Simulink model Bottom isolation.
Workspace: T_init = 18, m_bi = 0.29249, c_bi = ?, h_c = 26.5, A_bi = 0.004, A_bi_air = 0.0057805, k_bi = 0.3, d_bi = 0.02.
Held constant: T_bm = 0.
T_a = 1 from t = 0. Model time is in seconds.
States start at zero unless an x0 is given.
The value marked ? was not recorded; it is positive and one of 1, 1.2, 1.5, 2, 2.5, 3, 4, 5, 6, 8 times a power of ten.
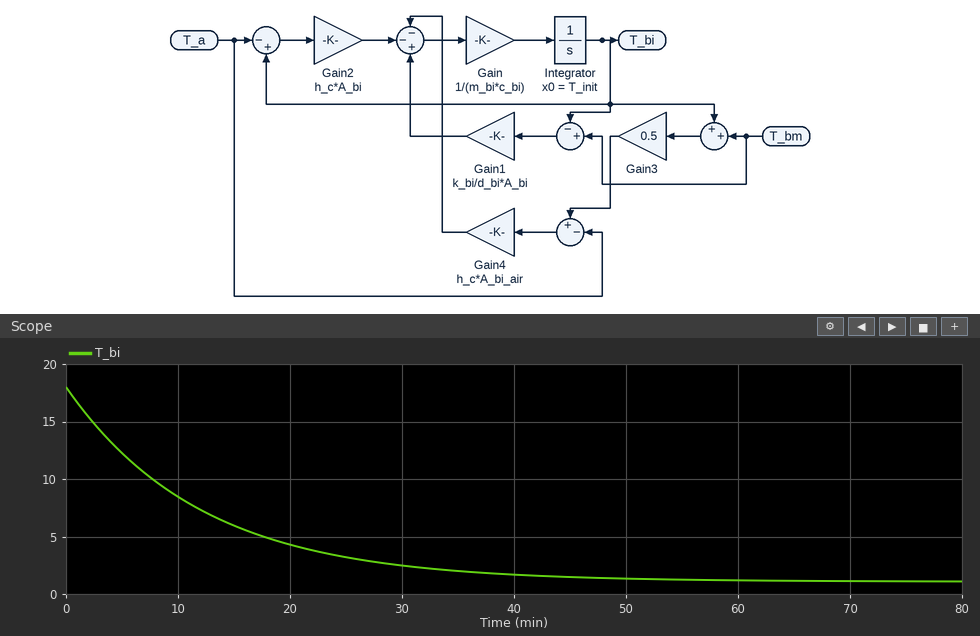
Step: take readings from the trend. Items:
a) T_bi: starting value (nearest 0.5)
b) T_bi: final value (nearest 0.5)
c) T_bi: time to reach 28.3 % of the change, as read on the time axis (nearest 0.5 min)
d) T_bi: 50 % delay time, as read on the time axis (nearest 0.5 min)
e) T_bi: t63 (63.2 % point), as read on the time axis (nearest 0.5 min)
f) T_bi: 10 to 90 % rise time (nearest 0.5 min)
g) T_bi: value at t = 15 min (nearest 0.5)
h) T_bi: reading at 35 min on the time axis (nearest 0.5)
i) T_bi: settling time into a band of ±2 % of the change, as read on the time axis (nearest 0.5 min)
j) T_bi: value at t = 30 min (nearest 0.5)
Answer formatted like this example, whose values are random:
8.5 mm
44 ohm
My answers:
18.0
1.0
4.0 min
8.5 min
12.0 min
26.5 min
6.0
2.0
47.0 min
2.5
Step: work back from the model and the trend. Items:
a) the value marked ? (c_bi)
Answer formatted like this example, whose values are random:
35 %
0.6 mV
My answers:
600
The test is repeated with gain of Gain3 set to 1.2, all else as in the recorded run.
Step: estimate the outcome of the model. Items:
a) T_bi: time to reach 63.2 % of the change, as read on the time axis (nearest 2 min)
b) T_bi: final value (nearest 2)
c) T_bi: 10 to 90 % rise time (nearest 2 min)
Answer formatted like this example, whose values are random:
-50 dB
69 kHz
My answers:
8 min
0
18 min
